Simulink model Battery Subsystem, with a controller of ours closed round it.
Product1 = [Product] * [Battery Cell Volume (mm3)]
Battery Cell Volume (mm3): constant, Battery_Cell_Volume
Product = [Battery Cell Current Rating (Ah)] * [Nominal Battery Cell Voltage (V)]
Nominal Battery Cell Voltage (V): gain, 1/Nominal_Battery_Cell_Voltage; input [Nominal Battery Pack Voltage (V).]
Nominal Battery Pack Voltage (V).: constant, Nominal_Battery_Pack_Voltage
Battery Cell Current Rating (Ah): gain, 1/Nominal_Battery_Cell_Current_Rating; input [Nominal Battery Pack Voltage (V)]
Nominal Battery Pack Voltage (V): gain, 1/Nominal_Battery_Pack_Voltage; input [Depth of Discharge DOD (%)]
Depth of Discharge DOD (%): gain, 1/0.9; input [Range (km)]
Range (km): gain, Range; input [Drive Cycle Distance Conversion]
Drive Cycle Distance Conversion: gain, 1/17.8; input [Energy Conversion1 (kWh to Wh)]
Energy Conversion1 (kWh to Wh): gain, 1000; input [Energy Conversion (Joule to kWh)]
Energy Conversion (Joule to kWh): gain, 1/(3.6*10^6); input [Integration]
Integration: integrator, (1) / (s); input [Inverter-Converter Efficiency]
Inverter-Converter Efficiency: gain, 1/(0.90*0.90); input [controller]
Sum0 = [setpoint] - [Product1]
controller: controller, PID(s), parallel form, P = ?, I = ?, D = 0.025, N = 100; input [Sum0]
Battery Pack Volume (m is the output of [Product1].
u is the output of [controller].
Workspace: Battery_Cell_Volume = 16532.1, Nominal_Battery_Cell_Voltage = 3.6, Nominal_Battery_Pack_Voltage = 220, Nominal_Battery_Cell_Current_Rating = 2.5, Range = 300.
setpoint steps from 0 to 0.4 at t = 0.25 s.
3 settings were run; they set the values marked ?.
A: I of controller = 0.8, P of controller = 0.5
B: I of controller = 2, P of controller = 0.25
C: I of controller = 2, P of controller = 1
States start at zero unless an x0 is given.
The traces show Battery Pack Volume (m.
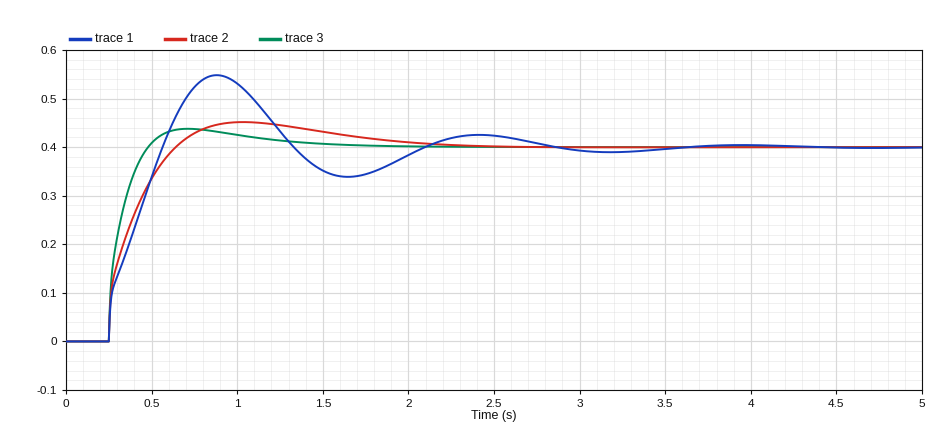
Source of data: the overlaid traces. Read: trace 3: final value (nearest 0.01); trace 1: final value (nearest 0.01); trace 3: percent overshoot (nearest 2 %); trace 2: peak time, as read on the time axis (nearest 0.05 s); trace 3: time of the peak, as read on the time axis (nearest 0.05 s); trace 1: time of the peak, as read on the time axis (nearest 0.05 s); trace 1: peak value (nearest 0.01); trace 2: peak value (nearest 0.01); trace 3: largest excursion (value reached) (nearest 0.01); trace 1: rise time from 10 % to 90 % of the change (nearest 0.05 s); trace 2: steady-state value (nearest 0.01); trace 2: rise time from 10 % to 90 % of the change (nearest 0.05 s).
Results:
0.40
0.40
10 %
1.05 s
0.70 s
0.90 s
0.55
0.45
0.44
0.25 s
0.40
0.30 s
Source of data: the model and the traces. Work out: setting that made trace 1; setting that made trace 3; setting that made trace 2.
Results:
B
C
A
